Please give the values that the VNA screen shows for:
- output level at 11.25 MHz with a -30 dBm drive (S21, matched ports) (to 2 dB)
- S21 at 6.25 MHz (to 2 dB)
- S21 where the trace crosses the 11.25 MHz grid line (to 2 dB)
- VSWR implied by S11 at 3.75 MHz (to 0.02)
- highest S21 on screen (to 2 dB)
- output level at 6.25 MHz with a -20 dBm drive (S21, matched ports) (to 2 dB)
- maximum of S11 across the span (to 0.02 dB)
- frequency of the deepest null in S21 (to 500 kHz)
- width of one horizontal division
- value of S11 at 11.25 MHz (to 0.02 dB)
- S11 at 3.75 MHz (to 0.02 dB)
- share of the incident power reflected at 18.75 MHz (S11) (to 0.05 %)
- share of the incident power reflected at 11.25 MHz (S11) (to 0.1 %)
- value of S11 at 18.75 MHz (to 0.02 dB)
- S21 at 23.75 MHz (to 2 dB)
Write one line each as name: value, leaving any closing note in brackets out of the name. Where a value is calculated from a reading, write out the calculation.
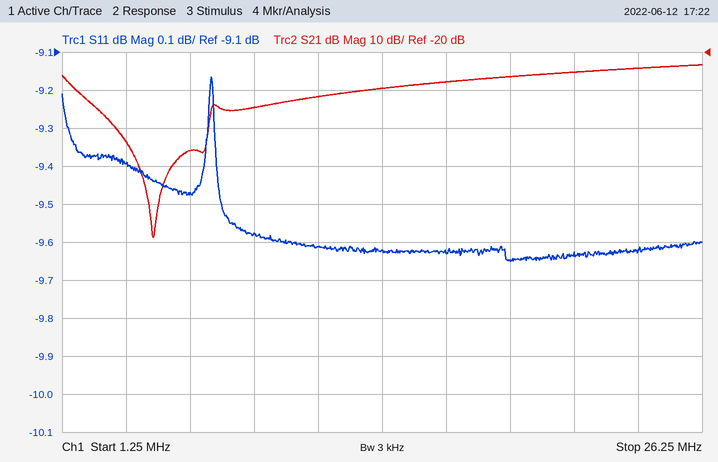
output level at 11.25 MHz with a -30 dBm drive (S21, matched ports): -30 dBm + (-32 dB) = -62 dBm
S21 at 6.25 MHz: -46 dB
S21 where the trace crosses the 11.25 MHz grid line: -32 dB
VSWR implied by S11 at 3.75 MHz: |Γ| = 10^(-9.4/20) = 0.3388; VSWR = (1 + 0.3388)/(1 − 0.3388) ≈ 2.03, so 2.02 to the nearest 0.02
highest S21 on screen: -24 dB
output level at 6.25 MHz with a -20 dBm drive (S21, matched ports): -20 dBm + (-46 dB) = -66 dBm
maximum of S11 across the span: -9.16 dB
frequency of the deepest null in S21: 5.0 MHz
width of one horizontal division: 2.5 MHz
value of S11 at 11.25 MHz: -9.62 dB
S11 at 3.75 MHz: -9.40 dB
share of the incident power reflected at 18.75 MHz (S11): 10^(-9.64/10) ≈ 10.9 %, so 10.85 % to the nearest 0.05 %
share of the incident power reflected at 11.25 MHz (S11): 10^(-9.62/10) ≈ 10.9 %
value of S11 at 18.75 MHz: -9.64 dB
S21 at 23.75 MHz: -24 dB
